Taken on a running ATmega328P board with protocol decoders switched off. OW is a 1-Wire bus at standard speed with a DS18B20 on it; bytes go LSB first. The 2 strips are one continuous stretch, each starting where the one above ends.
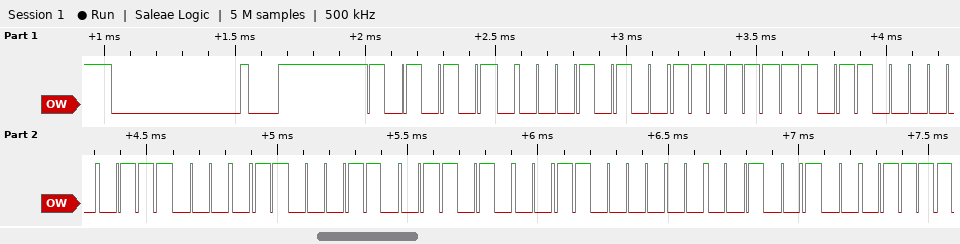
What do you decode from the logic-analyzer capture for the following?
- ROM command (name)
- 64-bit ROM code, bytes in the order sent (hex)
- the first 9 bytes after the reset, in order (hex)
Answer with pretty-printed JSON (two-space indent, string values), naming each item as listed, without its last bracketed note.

{
  "ROM command": "Match ROM",
  "64-bit ROM code, bytes in the order sent": "28 FF 06 0E 63 16 03 24",
  "the first 9 bytes after the reset, in order": "55 28 FF 06 0E 63 16 03 24"
}
